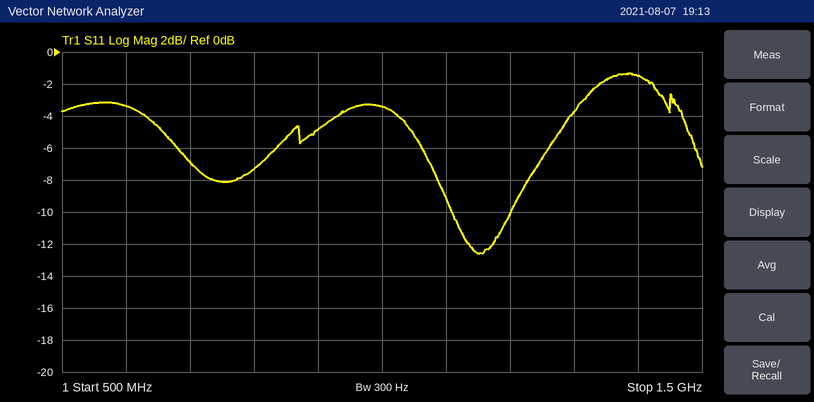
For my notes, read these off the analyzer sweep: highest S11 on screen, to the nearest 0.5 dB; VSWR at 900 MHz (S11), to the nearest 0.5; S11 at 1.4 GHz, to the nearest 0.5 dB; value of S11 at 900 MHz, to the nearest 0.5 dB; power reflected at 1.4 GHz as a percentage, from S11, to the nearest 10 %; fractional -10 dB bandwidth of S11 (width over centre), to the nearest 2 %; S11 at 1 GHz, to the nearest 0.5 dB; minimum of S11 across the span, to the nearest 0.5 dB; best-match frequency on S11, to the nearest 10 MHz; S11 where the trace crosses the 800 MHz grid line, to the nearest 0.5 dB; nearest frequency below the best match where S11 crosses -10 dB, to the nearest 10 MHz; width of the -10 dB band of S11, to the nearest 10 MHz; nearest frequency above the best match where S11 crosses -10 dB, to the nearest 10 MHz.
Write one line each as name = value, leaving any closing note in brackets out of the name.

highest S11 on screen, to the nearest 0.5 dB = -1.5 dB
VSWR at 900 MHz (S11), to the nearest 0.5 = 3.5
S11 at 1.4 GHz, to the nearest 0.5 dB = -1.5 dB
value of S11 at 900 MHz, to the nearest 0.5 dB = -5.0 dB
power reflected at 1.4 GHz as a percentage, from S11, to the nearest 10 % = 70 %
fractional -10 dB bandwidth of S11 (width over centre), to the nearest 2 % = 8 %
S11 at 1 GHz, to the nearest 0.5 dB = -3.5 dB
minimum of S11 across the span, to the nearest 0.5 dB = -12.5 dB
best-match frequency on S11, to the nearest 10 MHz = 1.15 GHz
S11 where the trace crosses the 800 MHz grid line, to the nearest 0.5 dB = -7.5 dB
nearest frequency below the best match where S11 crosses -10 dB, to the nearest 10 MHz = 1.11 GHz
width of the -10 dB band of S11, to the nearest 10 MHz = 90 MHz
nearest frequency above the best match where S11 crosses -10 dB, to the nearest 10 MHz = 1.20 GHz
